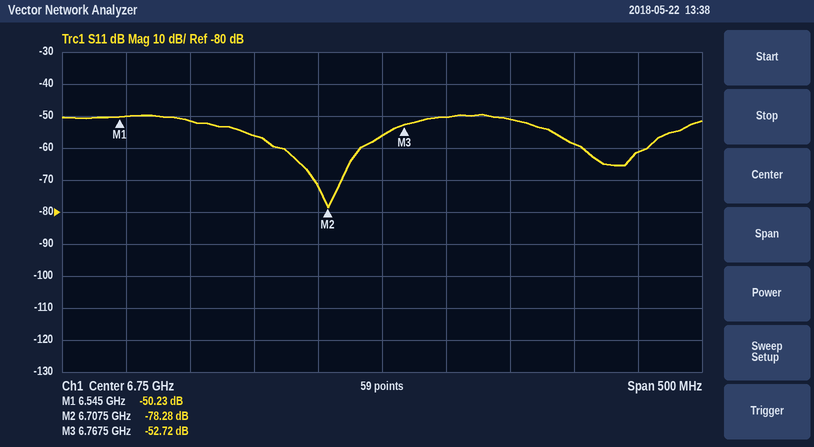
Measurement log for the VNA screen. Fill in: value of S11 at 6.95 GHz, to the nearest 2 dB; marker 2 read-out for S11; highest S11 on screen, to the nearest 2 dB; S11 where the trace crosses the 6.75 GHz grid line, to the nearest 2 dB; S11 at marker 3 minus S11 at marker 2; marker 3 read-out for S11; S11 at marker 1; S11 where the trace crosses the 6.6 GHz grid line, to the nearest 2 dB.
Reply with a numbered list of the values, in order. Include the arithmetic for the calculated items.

1. -62 dB
2. -78.28 dB
3. -50 dB
4. -56 dB
5. -52.72 − (-78.28) = 25.56 dB
6. -52.72 dB
7. -50.23 dB
8. -52 dB
